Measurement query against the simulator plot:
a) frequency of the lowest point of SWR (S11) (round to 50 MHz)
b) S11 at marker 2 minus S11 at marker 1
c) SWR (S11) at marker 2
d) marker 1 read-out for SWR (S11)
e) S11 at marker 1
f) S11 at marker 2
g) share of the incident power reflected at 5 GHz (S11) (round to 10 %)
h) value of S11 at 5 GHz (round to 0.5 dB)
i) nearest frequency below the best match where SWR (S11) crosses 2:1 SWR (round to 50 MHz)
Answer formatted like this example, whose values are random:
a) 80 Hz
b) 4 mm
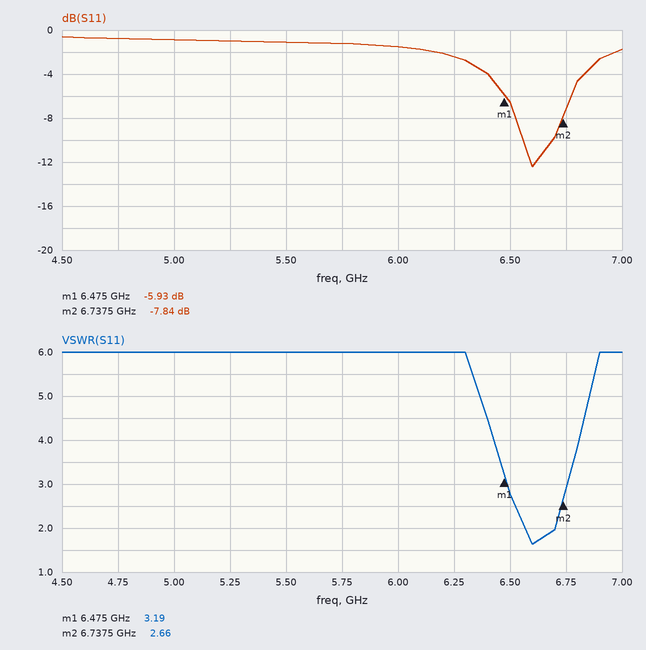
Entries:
a) 6.60 GHz
b) -1.91 dB
c) 2.66
d) 3.19
e) -5.93 dB
f) -7.84 dB
g) 80 %
h) -1.0 dB
i) 6.55 GHz
